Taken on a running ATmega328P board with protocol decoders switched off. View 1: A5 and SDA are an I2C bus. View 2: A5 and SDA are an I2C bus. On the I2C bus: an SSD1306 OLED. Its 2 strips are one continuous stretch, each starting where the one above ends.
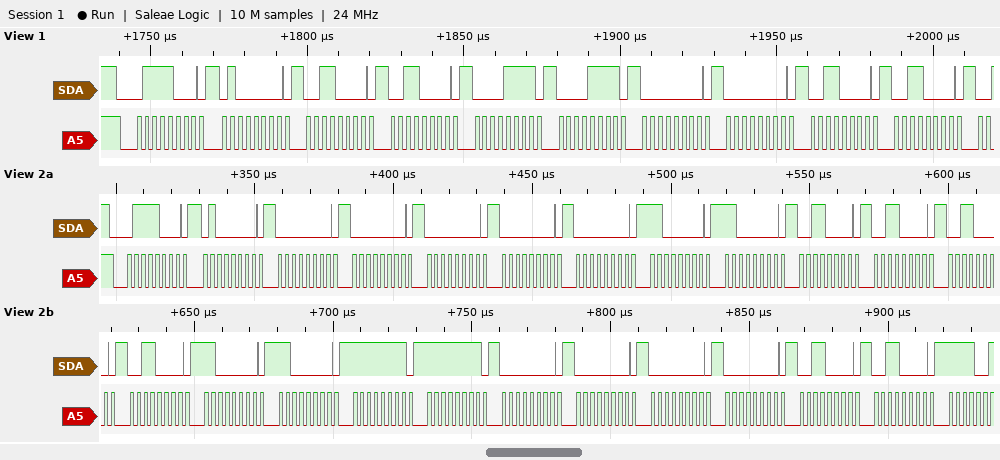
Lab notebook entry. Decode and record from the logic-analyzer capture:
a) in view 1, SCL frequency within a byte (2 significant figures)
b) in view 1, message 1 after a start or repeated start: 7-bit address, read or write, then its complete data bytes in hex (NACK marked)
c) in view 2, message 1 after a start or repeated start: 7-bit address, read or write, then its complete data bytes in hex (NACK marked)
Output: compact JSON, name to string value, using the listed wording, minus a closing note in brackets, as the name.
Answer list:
{"in view 1, SCL frequency within a byte": "400 kHz", "in view 1, message 1 after a start or repeated start: 7-bit address, read or write, then its complete data bytes in hex": "0x3C write: 40 30 30 0F 0F 00 00 30 30", "in view 2, message 1 after a start or repeated start: 7-bit address, read or write, then its complete data bytes in hex": "0x3C write: 40 00 00 00 00 00 C0 C0 30 30 30 30 C0 C0 FF FF 00 00 00 00 30 30"}
